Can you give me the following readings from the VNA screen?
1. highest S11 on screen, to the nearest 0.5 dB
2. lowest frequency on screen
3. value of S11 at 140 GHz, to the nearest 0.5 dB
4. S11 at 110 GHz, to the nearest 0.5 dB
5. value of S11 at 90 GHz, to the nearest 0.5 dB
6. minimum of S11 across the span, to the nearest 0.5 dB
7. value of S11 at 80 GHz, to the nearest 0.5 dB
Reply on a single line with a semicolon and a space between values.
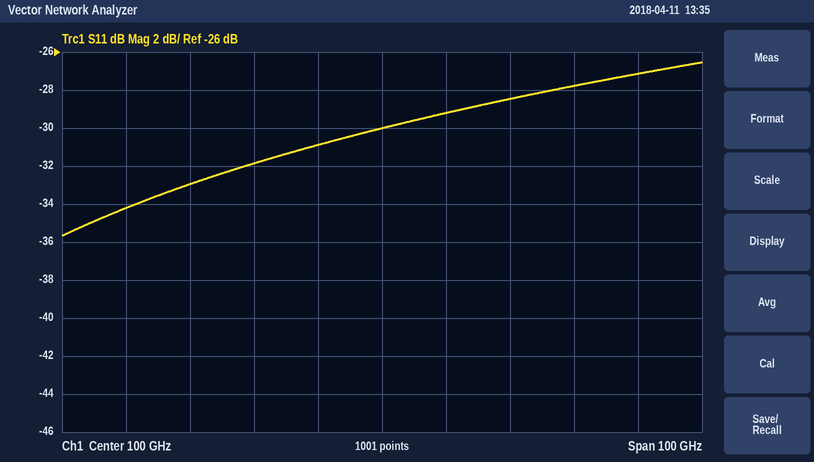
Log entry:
-26.5 dB; 50 GHz; -27.0 dB; -29.0 dB; -31.0 dB; -35.5 dB; -32.0 dB
